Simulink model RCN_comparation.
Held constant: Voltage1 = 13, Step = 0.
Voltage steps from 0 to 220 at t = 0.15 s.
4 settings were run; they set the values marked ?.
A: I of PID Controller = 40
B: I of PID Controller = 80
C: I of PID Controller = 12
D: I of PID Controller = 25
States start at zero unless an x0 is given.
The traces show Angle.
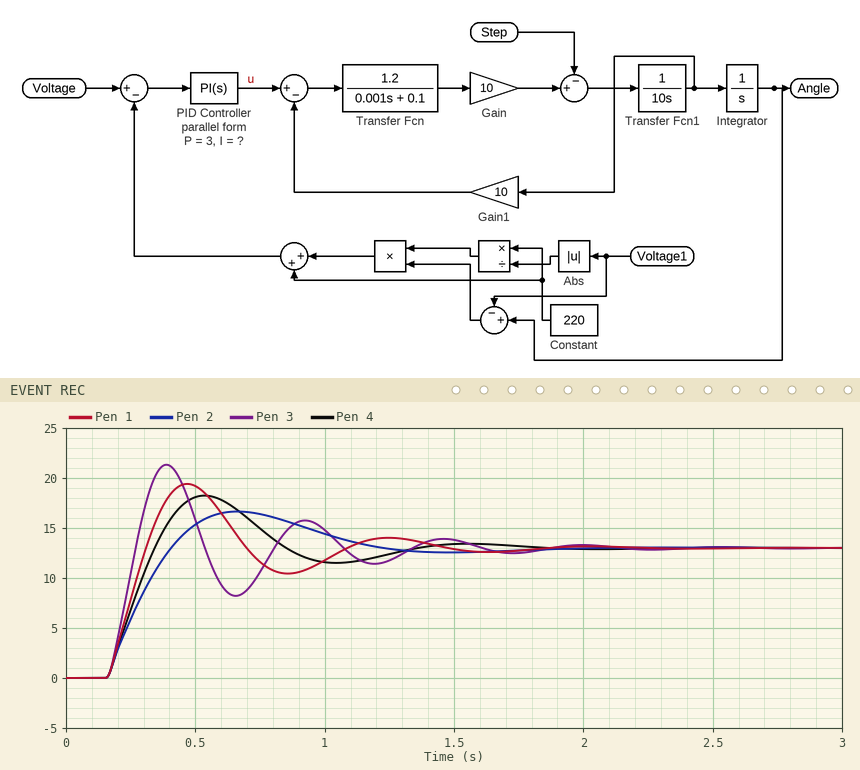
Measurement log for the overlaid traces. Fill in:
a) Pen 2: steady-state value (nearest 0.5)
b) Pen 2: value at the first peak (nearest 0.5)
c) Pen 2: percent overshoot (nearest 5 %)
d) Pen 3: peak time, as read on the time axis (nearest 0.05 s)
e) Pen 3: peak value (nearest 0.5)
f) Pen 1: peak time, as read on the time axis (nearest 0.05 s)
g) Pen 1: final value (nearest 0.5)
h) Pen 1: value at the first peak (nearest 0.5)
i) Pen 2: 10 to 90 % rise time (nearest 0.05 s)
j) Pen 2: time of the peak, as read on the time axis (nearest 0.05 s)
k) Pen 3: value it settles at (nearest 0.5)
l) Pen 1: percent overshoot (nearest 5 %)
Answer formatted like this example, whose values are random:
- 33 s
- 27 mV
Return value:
- 13.0
- 16.5
- 30 %
- 0.40 s
- 21.5
- 0.45 s
- 13.0
- 19.5
- 0.20 s
- 0.65 s
- 13.0
- 50 %
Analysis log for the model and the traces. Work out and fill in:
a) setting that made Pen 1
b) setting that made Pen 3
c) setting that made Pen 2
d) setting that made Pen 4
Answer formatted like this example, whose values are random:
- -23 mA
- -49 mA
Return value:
- A
- B
- C
- D
